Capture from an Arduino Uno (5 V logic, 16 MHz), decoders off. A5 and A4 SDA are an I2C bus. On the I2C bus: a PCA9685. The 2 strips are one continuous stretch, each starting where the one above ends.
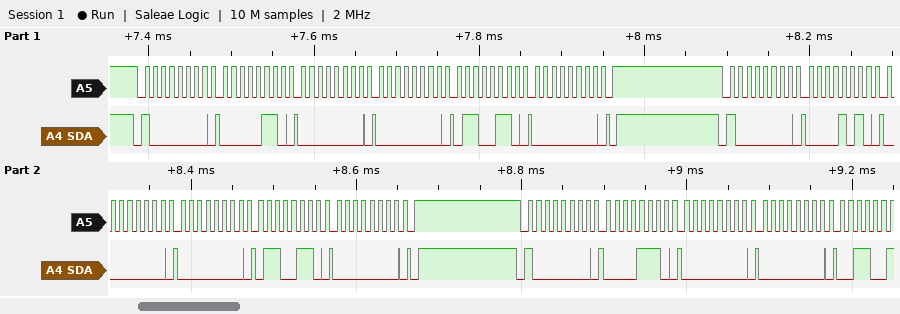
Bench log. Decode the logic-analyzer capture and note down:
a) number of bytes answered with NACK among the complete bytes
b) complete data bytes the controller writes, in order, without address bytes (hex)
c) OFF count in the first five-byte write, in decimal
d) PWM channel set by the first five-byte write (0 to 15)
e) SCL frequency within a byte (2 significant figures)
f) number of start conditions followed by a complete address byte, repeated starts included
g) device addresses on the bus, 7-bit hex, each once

0
06 00 00 66 00 0A 00 00 66 00 0E 00 00
102
0
100 kHz
3
0x40
